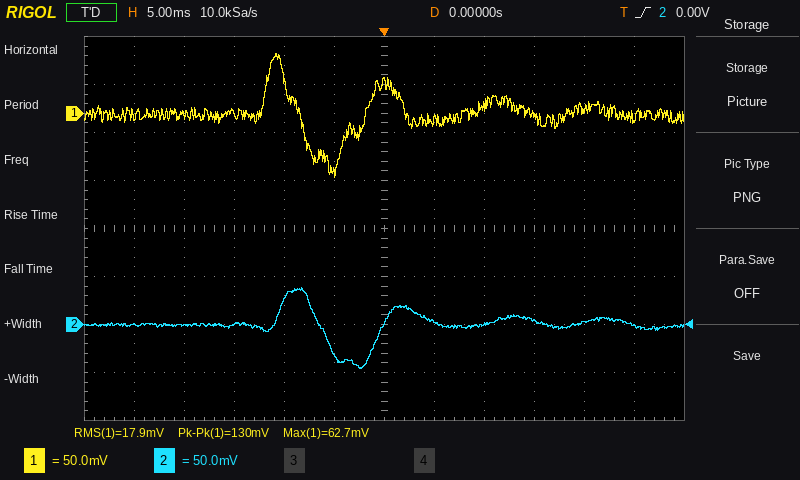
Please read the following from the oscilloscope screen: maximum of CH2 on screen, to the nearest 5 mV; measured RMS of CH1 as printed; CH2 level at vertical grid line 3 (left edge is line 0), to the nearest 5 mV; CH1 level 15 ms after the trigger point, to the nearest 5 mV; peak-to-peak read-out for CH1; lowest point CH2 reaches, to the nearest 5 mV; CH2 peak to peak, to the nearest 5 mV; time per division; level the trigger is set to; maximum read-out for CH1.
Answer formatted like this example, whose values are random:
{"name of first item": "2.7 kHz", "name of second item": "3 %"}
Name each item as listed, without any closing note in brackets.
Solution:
{"maximum of CH2 on screen, to the nearest 5 mV": "40 mV", "measured RMS of CH1 as printed": "17.9 mV", "CH2 level at vertical grid line 3 (left edge is line 0), to the nearest 5 mV": "0 mV", "CH1 level 15 ms after the trigger point, to the nearest 5 mV": "0 mV", "peak-to-peak read-out for CH1": "130 mV", "lowest point CH2 reaches, to the nearest 5 mV": "-45 mV", "CH2 peak to peak, to the nearest 5 mV": "85 mV", "time per division": "5 ms", "level the trigger is set to": "0.00 V", "maximum read-out for CH1": "62.7 mV"}
